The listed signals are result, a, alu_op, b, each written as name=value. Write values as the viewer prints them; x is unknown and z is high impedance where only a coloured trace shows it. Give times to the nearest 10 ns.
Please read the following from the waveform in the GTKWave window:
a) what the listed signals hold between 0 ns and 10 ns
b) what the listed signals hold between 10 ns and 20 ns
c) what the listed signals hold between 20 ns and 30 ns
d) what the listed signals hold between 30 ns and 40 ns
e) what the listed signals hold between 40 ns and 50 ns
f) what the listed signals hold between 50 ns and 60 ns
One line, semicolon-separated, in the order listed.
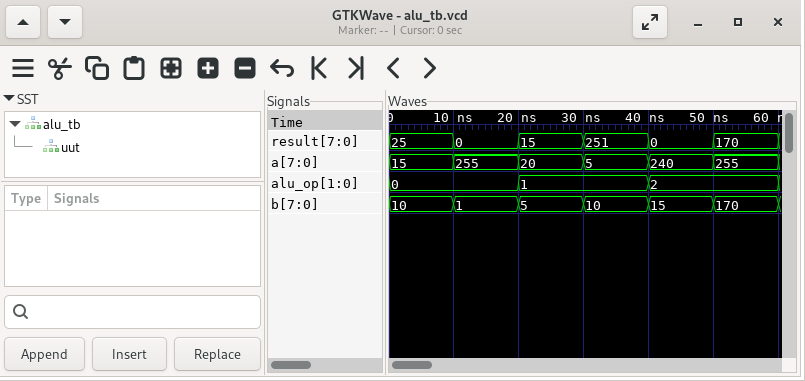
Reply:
result=25, a=15, alu_op=0, b=10; result=0, a=255, alu_op=0, b=1; result=15, a=20, alu_op=1, b=5; result=251, a=5, alu_op=1, b=10; result=0, a=240, alu_op=2, b=15; result=170, a=255, alu_op=2, b=170
